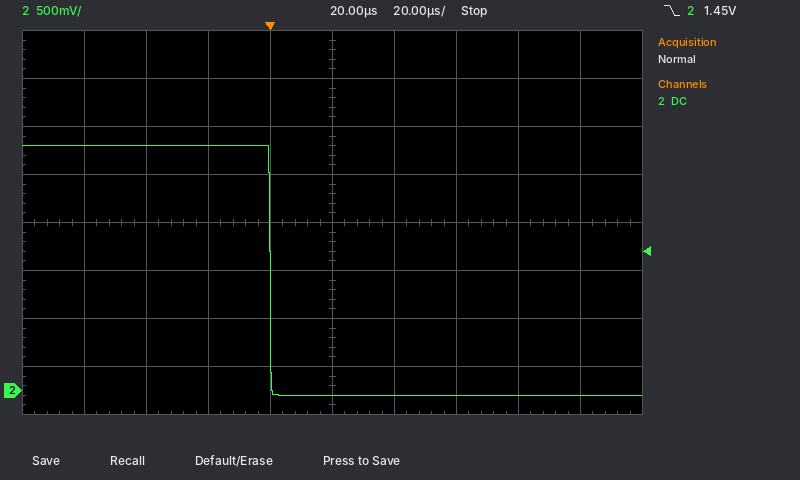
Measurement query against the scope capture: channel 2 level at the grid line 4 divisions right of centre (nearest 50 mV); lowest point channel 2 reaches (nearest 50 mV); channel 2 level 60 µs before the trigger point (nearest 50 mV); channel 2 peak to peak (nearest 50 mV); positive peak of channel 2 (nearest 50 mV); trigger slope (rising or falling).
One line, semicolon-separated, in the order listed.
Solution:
-50 mV; -50 mV; 2.55 V; 2.60 V; 2.55 V; falling
